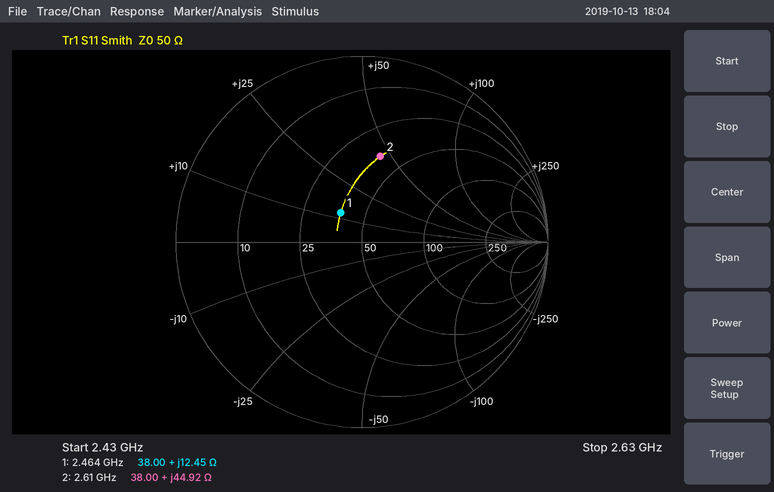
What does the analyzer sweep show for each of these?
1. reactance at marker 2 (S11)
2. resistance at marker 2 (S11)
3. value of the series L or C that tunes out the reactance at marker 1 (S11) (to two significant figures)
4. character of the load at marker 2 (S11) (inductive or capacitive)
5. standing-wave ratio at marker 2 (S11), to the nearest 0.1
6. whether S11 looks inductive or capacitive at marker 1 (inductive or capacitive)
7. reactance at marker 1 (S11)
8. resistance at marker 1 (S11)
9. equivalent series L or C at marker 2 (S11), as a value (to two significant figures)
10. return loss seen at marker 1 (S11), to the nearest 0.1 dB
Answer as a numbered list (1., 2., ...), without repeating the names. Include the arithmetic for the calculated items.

1. +44.92 Ω
2. 38.00 Ω
3. C = 1/(2π × 2.464 GHz × 12.45 Ω) ≈ 5.2 pF
4. inductive
5. 2.8
6. inductive
7. +12.45 Ω
8. 38.00 Ω
9. L = 44.92 Ω/(2π × 2.61 GHz) ≈ 2.7 nH
10. 14.2 dB
